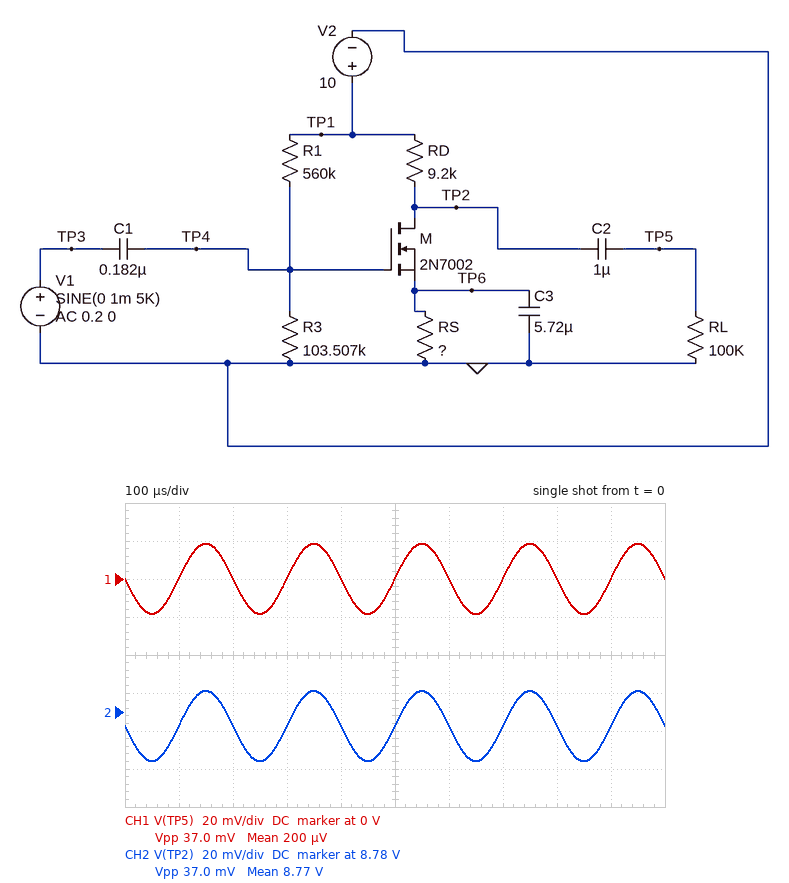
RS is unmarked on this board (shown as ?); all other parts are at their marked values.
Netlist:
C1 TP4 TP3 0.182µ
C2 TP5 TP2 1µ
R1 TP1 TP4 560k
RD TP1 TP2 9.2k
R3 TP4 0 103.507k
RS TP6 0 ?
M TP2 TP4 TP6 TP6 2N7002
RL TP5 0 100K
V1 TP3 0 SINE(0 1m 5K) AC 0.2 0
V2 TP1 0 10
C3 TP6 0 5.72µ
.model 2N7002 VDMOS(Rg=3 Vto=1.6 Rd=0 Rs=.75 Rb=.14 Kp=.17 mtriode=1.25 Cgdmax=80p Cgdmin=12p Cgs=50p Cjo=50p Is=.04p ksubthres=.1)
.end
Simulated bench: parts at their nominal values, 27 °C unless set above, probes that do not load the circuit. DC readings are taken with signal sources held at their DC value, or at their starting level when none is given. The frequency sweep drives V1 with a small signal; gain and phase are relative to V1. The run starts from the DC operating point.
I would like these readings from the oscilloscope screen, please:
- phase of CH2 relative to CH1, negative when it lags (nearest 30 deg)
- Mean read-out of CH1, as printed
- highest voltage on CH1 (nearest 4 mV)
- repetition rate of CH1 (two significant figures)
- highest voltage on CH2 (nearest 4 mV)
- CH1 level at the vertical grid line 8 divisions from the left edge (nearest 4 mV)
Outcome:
0 deg
200 µV
20 mV
5.0 kHz
8.792 V
0 V
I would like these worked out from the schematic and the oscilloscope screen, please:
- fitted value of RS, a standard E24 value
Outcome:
240 Ω
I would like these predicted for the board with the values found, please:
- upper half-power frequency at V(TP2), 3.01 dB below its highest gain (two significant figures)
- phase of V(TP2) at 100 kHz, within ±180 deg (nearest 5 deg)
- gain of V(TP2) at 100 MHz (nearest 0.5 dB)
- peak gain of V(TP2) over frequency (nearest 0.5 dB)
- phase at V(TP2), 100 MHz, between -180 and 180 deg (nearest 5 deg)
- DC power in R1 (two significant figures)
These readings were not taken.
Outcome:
630 kHz
170 deg
-5.5 dB
25.5 dB
5 deg
130 µW
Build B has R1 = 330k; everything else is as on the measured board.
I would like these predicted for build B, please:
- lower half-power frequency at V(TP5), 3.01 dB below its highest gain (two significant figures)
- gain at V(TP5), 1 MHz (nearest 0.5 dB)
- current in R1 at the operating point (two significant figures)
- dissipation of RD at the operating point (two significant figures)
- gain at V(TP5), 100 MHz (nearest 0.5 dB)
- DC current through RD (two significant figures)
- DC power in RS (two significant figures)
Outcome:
86 MHz
-34.5 dB
23 µA
10 mW
-8.5 dB
1.1 mA
270 µW
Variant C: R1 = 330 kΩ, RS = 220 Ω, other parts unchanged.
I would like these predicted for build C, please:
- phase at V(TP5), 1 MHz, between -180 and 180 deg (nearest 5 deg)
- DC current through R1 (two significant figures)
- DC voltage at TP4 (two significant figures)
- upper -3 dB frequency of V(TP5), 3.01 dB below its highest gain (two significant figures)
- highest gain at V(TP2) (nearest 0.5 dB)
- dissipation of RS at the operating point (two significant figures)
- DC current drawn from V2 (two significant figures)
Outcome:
165 deg
23 µA
2.4 V
950 MHz
-6.5 dB
250 µW
1.1 mA
